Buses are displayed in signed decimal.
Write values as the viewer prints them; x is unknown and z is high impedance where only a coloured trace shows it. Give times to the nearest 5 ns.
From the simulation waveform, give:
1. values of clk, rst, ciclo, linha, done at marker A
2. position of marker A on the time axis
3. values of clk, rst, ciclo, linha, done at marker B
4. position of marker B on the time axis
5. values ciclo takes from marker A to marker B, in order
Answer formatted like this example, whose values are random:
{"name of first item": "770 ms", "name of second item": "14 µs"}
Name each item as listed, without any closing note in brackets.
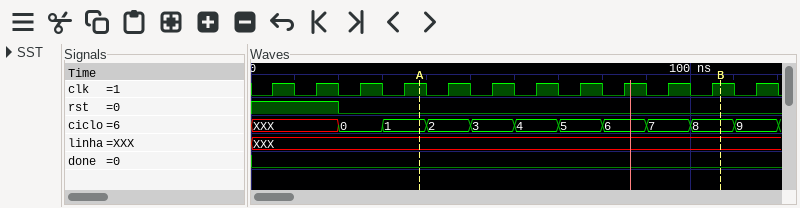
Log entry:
{"values of clk, rst, ciclo, linha, done at marker A": "clk=1, rst=0, ciclo=1, linha=XXX, done=0", "position of marker A on the time axis": "40 ns", "values of clk, rst, ciclo, linha, done at marker B": "clk=1, rst=0, ciclo=8, linha=XXX, done=0", "position of marker B on the time axis": "105 ns", "values ciclo takes from marker A to marker B, in order": "1, 2, 3, 4, 5, 6, 7, 8"}
